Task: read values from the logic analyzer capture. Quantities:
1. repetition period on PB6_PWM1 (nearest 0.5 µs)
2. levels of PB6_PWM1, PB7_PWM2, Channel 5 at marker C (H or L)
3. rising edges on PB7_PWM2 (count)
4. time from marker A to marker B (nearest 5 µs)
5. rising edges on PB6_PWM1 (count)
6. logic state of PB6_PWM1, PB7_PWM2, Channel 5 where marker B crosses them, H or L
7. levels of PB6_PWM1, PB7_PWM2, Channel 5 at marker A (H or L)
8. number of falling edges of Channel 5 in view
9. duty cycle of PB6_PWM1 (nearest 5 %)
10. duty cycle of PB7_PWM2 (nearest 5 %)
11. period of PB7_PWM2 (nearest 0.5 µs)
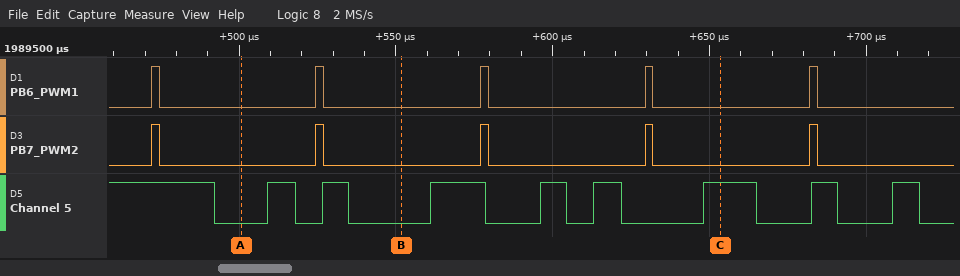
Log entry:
52.5 µs
PB6_PWM1=L, PB7_PWM2=L, Channel 5=H
5
50 µs
5
PB6_PWM1=L, PB7_PWM2=L, Channel 5=L
PB6_PWM1=L, PB7_PWM2=L, Channel 5=L
9
5 %
5 %
52.5 µs
